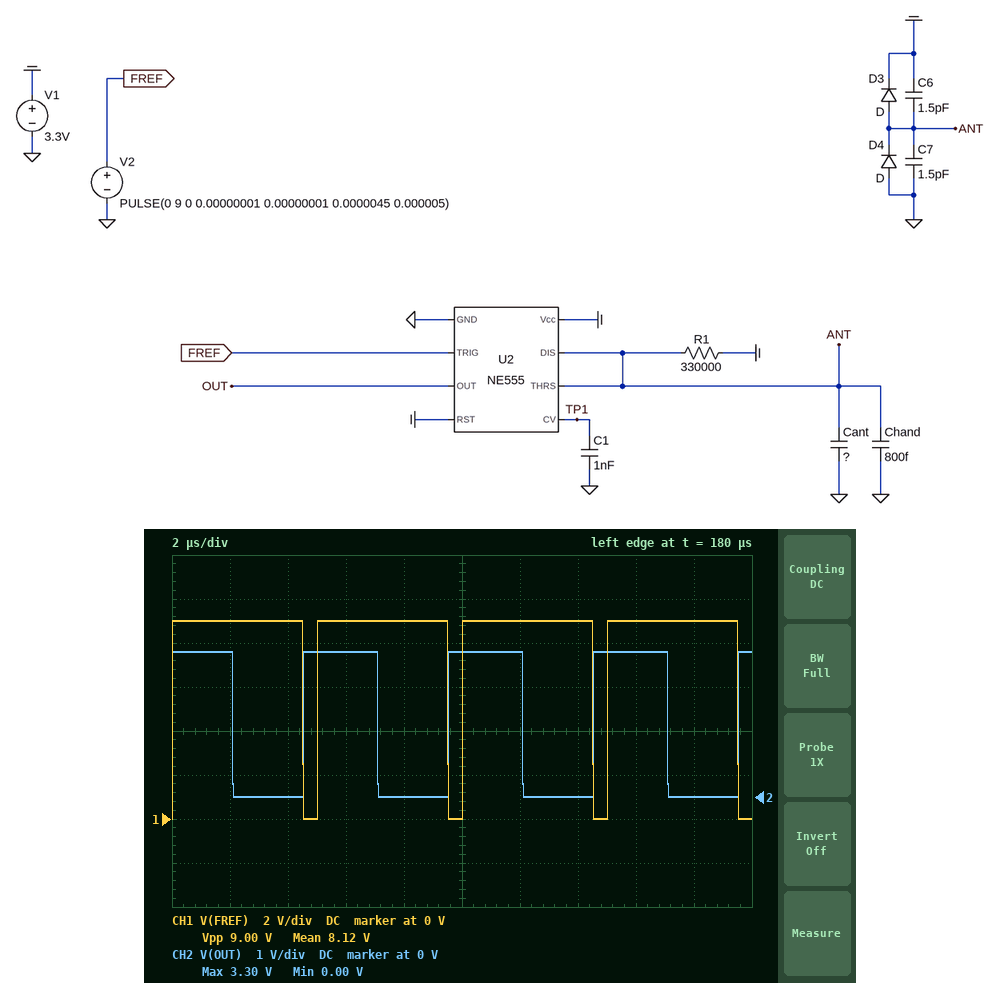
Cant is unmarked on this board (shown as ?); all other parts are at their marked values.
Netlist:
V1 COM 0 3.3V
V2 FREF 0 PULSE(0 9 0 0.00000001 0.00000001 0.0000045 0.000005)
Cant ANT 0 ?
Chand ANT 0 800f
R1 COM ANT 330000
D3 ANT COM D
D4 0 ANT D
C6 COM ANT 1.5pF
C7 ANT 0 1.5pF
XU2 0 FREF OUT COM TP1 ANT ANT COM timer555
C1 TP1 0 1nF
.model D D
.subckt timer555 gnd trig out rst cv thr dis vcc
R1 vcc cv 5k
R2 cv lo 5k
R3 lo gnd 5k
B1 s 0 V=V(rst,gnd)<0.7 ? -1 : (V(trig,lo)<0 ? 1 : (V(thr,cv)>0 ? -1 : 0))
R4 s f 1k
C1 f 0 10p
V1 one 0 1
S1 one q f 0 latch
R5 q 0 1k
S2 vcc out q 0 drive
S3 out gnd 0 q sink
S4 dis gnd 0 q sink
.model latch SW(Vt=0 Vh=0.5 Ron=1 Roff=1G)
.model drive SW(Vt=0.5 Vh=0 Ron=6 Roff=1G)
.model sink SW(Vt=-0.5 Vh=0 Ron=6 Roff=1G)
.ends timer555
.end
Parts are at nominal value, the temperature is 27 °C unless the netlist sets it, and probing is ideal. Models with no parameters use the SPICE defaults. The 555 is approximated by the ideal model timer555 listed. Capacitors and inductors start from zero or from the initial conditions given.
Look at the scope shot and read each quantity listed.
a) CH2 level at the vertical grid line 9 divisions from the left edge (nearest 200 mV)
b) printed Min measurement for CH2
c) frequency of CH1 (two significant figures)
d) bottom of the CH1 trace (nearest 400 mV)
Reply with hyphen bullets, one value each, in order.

- 0 V
- 0.00 V
- 200 kHz
- 0 V
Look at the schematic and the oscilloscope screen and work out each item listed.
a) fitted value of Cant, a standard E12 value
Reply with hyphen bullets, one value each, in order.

- 3.3 pF
